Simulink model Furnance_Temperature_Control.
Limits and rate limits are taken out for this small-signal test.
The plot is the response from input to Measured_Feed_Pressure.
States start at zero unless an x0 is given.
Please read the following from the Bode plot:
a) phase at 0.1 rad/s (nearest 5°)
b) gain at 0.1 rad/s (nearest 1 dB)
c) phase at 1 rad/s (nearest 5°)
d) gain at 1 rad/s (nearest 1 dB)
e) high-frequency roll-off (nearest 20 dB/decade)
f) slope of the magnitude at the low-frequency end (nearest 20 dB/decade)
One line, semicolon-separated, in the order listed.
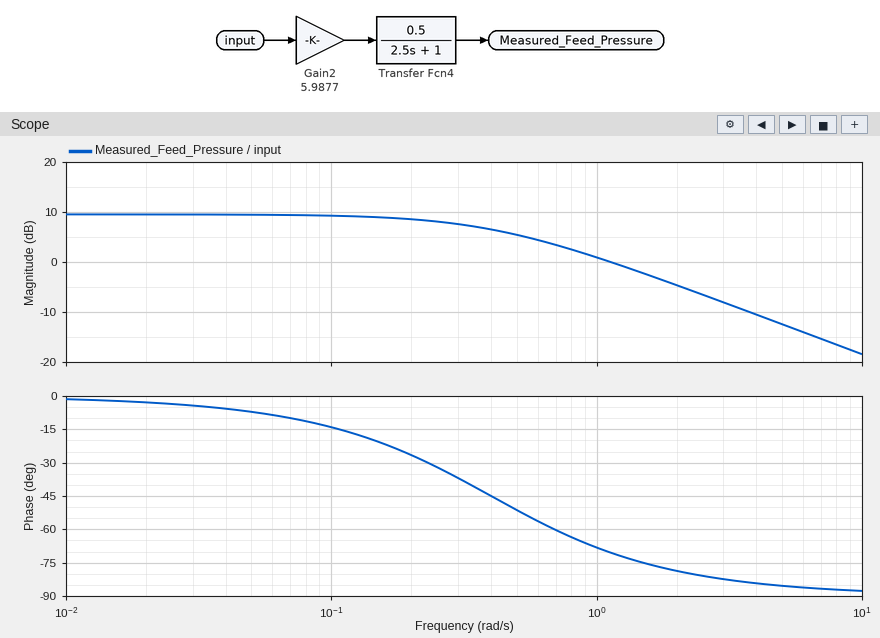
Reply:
-15°; 9 dB; -70°; 1 dB; -20 dB/decade; 0 dB/decade
